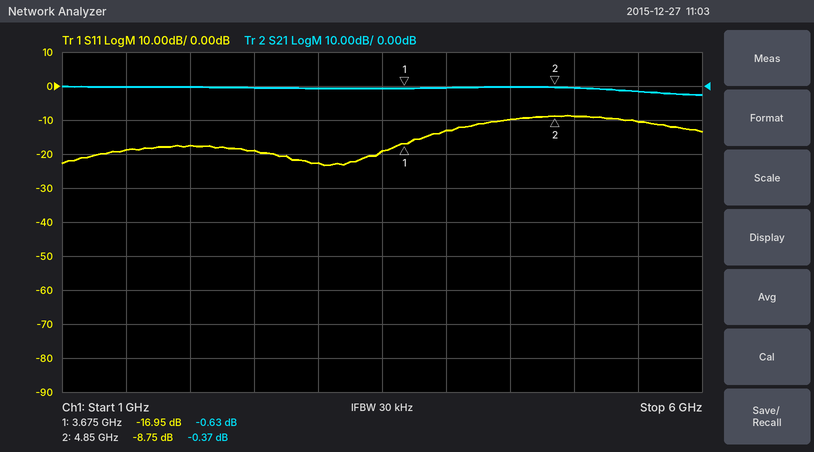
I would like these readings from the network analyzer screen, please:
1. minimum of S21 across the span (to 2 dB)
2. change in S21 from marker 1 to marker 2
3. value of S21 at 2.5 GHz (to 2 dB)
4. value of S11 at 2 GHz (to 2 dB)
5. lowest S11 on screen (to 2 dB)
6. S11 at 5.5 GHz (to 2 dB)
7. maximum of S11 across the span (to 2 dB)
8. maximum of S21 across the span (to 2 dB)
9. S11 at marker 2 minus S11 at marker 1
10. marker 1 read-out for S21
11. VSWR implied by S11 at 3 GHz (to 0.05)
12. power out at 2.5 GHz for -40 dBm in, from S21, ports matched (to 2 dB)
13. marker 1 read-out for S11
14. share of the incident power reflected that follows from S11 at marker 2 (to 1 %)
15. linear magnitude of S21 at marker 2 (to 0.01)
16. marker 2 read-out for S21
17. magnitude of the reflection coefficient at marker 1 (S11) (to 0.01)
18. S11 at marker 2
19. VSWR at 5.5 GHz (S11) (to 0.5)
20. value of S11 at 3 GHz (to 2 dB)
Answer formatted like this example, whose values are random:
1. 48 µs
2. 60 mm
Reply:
1. -2 dB
2. 0.26 dB
3. 0 dB
4. -18 dB
5. -24 dB
6. -10 dB
7. -8 dB
8. 0 dB
9. 8.20 dB
10. -0.63 dB
11. 1.15
12. -40 dBm
13. -16.95 dB
14. 13 %
15. 0.96
16. -0.37 dB
17. 0.14
18. -8.75 dB
19. 2.0
20. -22 dB
